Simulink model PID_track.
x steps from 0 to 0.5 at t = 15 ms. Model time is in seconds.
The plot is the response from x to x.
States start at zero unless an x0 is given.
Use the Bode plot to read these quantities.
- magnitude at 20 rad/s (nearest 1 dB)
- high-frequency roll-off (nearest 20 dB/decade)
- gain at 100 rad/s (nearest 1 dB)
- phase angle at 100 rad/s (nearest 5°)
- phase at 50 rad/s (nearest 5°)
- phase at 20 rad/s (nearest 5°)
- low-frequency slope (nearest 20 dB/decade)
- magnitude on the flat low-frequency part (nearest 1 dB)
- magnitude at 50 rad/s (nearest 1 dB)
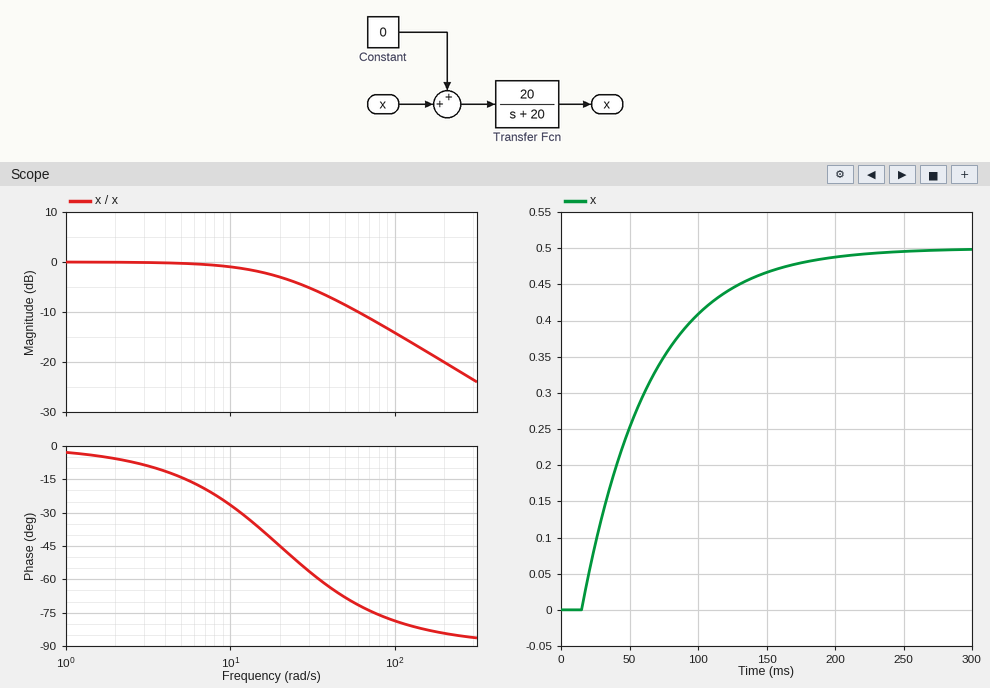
-3 dB
-20 dB/decade
-14 dB
-80°
-70°
-45°
0 dB/decade
0 dB
-9 dB
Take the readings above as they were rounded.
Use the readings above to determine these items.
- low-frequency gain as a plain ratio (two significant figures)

1.0
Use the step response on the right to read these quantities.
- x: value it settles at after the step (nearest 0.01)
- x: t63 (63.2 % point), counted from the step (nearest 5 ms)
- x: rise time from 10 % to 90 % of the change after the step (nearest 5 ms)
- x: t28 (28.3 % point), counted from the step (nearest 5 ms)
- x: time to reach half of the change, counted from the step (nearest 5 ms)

0.50
50 ms
110 ms
15 ms
35 ms
